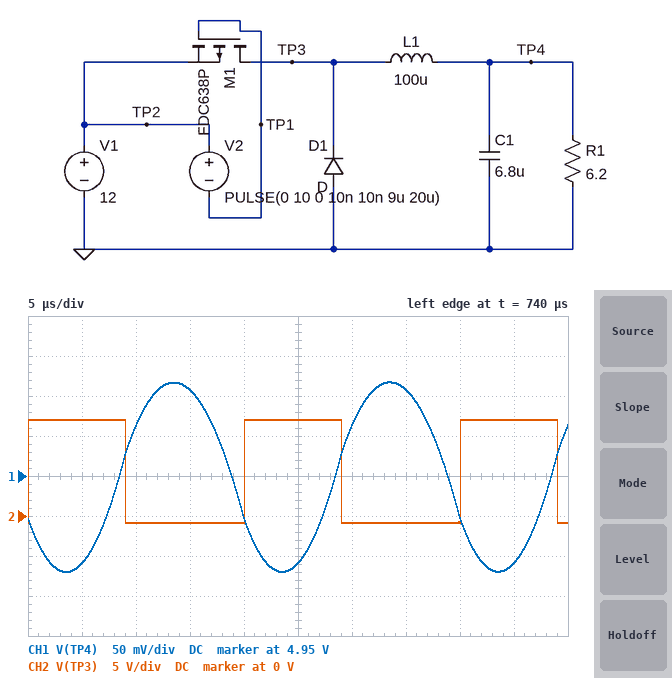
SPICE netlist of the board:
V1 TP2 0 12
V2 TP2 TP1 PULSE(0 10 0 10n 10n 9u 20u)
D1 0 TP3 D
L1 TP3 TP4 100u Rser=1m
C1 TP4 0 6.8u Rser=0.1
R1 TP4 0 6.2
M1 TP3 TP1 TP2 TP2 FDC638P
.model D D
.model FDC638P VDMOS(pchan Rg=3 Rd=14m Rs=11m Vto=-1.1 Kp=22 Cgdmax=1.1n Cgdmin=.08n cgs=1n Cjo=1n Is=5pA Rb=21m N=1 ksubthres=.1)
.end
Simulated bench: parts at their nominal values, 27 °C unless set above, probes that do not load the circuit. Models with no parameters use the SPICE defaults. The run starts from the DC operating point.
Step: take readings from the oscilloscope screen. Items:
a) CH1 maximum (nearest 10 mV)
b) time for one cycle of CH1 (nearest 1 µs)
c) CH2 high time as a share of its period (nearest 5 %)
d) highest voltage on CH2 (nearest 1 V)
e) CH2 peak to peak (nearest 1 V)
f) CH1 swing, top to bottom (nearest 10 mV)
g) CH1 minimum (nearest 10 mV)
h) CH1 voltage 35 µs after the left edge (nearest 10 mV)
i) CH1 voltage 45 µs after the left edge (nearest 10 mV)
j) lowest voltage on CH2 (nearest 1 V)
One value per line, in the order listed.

5.07 V
20 µs
45 %
12 V
13 V
240 mV
4.83 V
5.06 V
4.84 V
-1 V
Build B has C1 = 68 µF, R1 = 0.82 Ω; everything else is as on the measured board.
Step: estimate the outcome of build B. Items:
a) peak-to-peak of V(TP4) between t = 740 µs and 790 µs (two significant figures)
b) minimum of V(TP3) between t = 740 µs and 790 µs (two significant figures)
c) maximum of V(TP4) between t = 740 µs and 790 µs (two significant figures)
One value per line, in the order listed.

58 mV
-880 mV
4.9 V
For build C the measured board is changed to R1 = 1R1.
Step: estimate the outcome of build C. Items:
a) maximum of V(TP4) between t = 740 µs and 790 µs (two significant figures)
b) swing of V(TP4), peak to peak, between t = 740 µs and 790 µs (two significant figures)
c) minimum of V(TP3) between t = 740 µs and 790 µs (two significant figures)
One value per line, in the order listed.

5.0 V
210 mV
-870 mV
